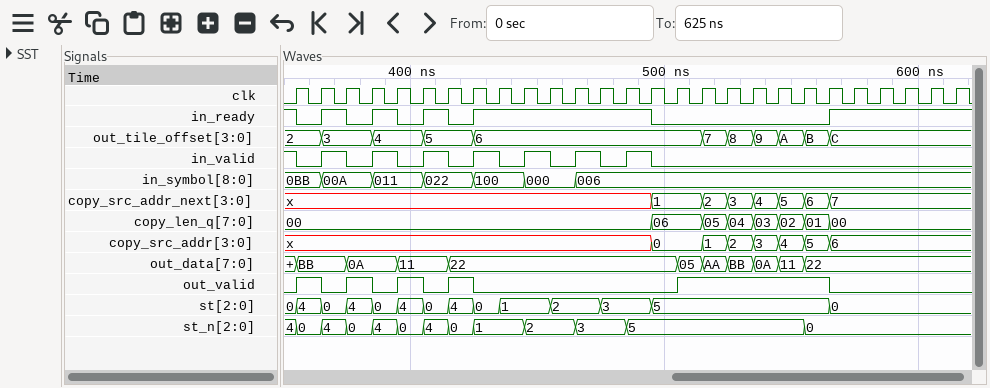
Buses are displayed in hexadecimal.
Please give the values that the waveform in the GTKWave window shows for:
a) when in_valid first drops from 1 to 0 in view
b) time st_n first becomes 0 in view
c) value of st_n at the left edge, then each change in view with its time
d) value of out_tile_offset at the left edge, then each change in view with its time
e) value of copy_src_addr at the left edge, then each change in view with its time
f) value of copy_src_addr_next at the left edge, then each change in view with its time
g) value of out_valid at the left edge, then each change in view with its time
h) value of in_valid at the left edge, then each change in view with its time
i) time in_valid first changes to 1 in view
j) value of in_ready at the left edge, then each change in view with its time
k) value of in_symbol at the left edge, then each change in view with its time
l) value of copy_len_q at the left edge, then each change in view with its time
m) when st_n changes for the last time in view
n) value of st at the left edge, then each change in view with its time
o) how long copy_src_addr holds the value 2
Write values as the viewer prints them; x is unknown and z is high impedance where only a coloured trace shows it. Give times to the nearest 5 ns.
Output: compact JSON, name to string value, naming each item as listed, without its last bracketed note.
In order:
{"when in_valid first drops from 1 to 0 in view": "355 ns", "time st_n first becomes 0 in view": "355 ns", "value of st_n at the left edge, then each change in view with its time": "4, 0 at 355 ns, 4 at 365 ns, 0 at 375 ns, 4 at 385 ns, 0 at 395 ns, 4 at 405 ns, 0 at 415 ns, 1 at 425 ns, 2 at 445 ns, 3 at 465 ns, 5 at 485 ns, 0 at 555 ns", "value of out_tile_offset at the left edge, then each change in view with its time": "2, 3 at 365 ns, 4 at 385 ns, 5 at 405 ns, 6 at 425 ns, 7 at 515 ns, 8 at 525 ns, 9 at 535 ns, A at 545 ns, B at 555 ns, C at 565 ns", "value of copy_src_addr at the left edge, then each change in view with its time": "x, 0 at 495 ns, 1 at 515 ns, 2 at 525 ns, 3 at 535 ns, 4 at 545 ns, 5 at 555 ns, 6 at 565 ns", "value of copy_src_addr_next at the left edge, then each change in view with its time": "x, 1 at 495 ns, 2 at 515 ns, 3 at 525 ns, 4 at 535 ns, 5 at 545 ns, 6 at 555 ns, 7 at 565 ns", "value of out_valid at the left edge, then each change in view with its time": "0, 1 at 355 ns, 0 at 365 ns, 1 at 375 ns, 0 at 385 ns, 1 at 395 ns, 0 at 405 ns, 1 at 415 ns, 0 at 425 ns, 1 at 505 ns, 0 at 565 ns", "value of in_valid at the left edge, then each change in view with its time": "1, 0 at 355 ns, 1 at 365 ns, 0 at 375 ns, 1 at 385 ns, 0 at 395 ns, 1 at 405 ns, 0 at 415 ns, 1 at 425 ns, 0 at 435 ns, 1 at 445 ns, 0 at 455 ns, 1 at 465 ns, 0 at 475 ns, 1 at 485 ns, 0 at 495 ns", "time in_valid first changes to 1 in view": "365 ns", "value of in_ready at the left edge, then each change in view with its time": "1, 0 at 355 ns, 1 at 365 ns, 0 at 375 ns, 1 at 385 ns, 0 at 395 ns, 1 at 405 ns, 0 at 415 ns, 1 at 425 ns, 0 at 495 ns, 1 at 565 ns", "value of in_symbol at the left edge, then each change in view with its time": "0BB, 00A at 365 ns, 011 at 385 ns, 022 at 405 ns, 100 at 425 ns, 000 at 445 ns, 006 at 465 ns", "value of copy_len_q at the left edge, then each change in view with its time": "00, 06 at 495 ns, 05 at 515 ns, 04 at 525 ns, 03 at 535 ns, 02 at 545 ns, 01 at 555 ns, 00 at 565 ns", "when st_n changes for the last time in view": "555 ns", "value of st at the left edge, then each change in view with its time": "0, 4 at 355 ns, 0 at 365 ns, 4 at 375 ns, 0 at 385 ns, 4 at 395 ns, 0 at 405 ns, 4 at 415 ns, 0 at 425 ns, 1 at 435 ns, 2 at 455 ns, 3 at 475 ns, 5 at 495 ns, 0 at 565 ns", "how long copy_src_addr holds the value 2": "10 ns"}
